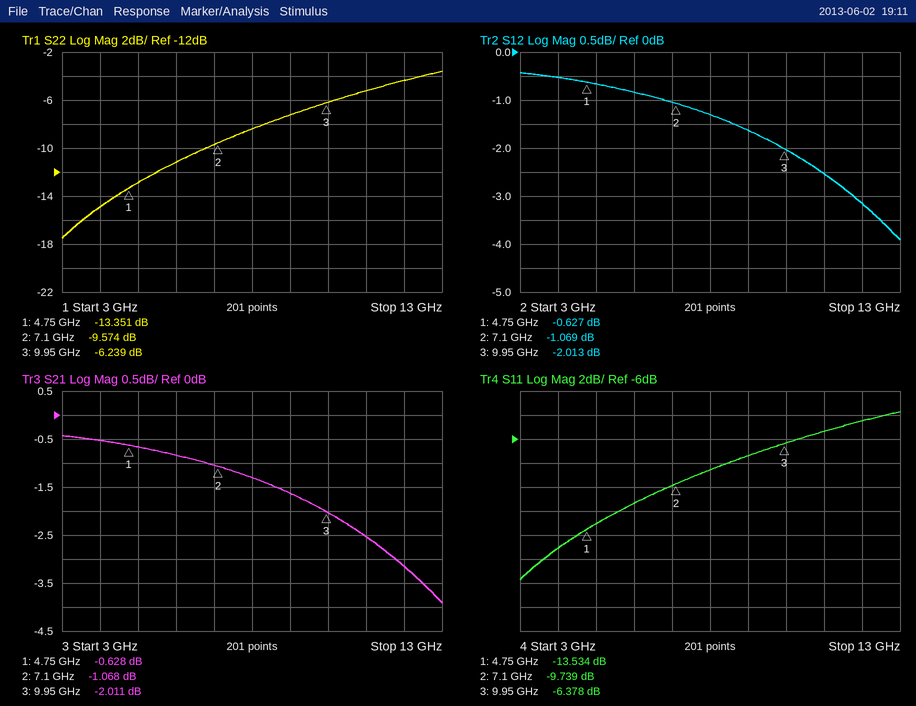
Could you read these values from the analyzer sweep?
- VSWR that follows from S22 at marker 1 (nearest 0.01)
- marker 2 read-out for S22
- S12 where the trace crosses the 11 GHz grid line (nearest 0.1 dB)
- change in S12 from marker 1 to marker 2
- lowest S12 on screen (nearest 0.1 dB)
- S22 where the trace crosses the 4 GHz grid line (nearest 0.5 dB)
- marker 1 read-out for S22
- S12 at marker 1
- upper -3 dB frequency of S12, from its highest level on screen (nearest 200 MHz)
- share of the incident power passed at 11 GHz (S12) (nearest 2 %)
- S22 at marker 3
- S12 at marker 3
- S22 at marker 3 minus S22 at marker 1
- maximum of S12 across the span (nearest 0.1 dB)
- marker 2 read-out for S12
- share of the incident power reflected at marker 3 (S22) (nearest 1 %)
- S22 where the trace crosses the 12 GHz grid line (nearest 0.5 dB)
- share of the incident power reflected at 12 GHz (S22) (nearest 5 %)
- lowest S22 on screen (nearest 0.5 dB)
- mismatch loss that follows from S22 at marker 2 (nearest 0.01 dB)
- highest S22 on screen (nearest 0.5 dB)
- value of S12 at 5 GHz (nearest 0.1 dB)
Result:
1.55
-9.574 dB
-2.5 dB
-0.442 dB
-3.9 dB
-15.0 dB
-13.351 dB
-0.627 dB
12.4 GHz
56 %
-6.239 dB
-2.013 dB
7.112 dB
-0.4 dB
-1.069 dB
24 %
-4.5 dB
35 %
-17.5 dB
0.51 dB
-3.5 dB
-0.7 dB
